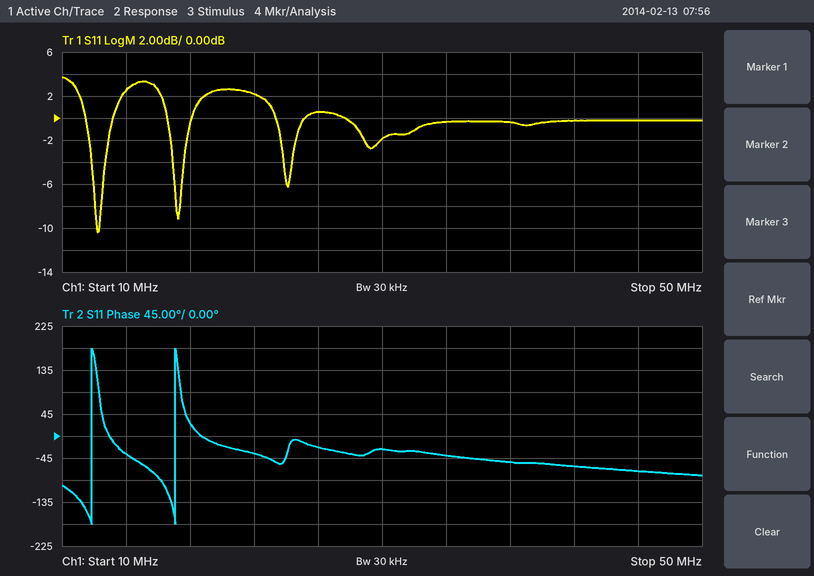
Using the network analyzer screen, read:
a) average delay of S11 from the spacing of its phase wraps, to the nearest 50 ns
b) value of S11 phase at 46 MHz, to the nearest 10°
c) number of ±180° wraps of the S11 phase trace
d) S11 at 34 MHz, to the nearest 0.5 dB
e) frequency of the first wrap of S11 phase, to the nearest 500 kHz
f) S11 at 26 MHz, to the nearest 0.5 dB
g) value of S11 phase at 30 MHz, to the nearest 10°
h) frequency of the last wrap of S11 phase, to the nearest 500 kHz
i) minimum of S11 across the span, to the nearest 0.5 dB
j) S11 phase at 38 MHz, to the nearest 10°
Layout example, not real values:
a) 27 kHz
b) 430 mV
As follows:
a) 200 ns
b) -70°
c) 2
d) -0.5 dB
e) 12.0 MHz
f) 0.5 dB
g) -30°
h) 17.0 MHz
i) -10.5 dB
j) -50°
